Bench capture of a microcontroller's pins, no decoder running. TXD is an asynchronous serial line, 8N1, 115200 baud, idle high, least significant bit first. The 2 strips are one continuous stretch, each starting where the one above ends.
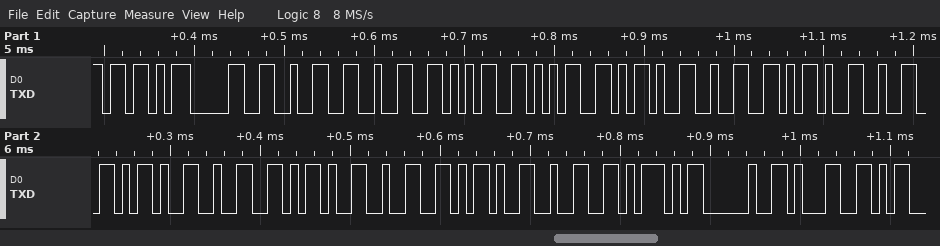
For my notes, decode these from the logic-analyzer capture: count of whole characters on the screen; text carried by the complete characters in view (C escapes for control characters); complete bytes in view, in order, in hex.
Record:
19
"[02255-2-2-2-2-2] 1"
5B 30 32 32 35 35 2D 32 2D 32 2D 32 2D 32 2D 32 5D 20 31
